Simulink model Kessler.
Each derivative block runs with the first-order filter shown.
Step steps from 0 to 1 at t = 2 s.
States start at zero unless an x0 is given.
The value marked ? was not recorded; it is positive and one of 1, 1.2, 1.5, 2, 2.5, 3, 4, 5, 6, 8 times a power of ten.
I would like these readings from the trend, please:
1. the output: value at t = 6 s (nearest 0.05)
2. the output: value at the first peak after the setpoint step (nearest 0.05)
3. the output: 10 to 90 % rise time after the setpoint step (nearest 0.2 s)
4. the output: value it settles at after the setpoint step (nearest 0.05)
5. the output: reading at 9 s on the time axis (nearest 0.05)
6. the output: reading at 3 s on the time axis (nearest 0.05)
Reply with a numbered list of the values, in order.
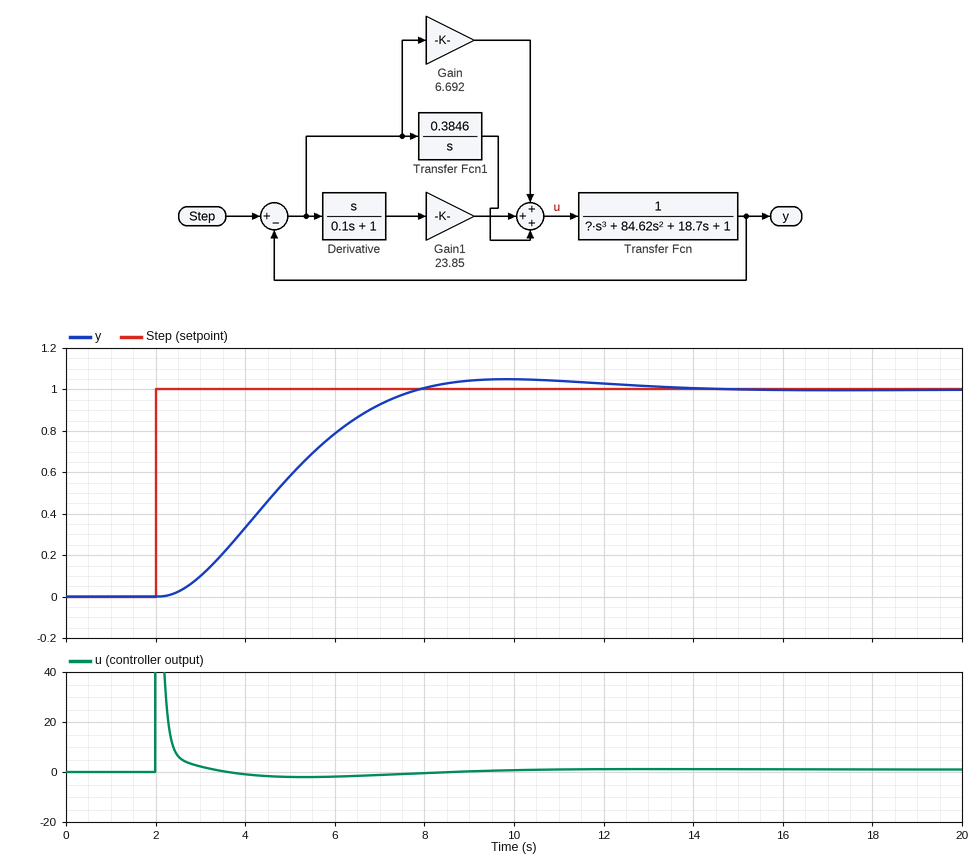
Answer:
1. 0.80
2. 1.05
3. 3.8 s
4. 1.00
5. 1.05
6. 0.10
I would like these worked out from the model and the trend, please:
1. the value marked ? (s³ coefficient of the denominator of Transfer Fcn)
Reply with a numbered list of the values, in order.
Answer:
1. 80
